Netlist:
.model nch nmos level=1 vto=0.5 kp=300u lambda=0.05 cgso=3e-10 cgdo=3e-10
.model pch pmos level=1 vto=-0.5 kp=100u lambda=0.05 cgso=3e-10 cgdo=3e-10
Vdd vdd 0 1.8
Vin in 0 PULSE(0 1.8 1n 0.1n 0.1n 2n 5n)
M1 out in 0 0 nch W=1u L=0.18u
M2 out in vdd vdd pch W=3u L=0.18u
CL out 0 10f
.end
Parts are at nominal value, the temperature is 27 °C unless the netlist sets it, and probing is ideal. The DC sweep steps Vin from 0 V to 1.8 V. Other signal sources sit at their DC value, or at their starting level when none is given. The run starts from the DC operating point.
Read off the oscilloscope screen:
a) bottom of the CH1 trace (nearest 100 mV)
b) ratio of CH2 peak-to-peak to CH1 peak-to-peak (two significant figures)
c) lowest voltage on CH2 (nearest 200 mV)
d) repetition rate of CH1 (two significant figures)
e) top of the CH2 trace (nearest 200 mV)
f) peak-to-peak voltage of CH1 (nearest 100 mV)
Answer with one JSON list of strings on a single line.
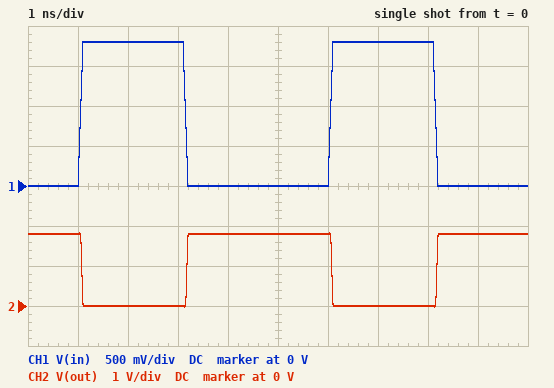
["0 V", "1.0", "0 V", "200 MHz", "1.8 V", "1.8 V"]
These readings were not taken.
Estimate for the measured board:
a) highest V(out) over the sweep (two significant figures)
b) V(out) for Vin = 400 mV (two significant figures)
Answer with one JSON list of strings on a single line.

["1.8 V", "1.8 V"]
